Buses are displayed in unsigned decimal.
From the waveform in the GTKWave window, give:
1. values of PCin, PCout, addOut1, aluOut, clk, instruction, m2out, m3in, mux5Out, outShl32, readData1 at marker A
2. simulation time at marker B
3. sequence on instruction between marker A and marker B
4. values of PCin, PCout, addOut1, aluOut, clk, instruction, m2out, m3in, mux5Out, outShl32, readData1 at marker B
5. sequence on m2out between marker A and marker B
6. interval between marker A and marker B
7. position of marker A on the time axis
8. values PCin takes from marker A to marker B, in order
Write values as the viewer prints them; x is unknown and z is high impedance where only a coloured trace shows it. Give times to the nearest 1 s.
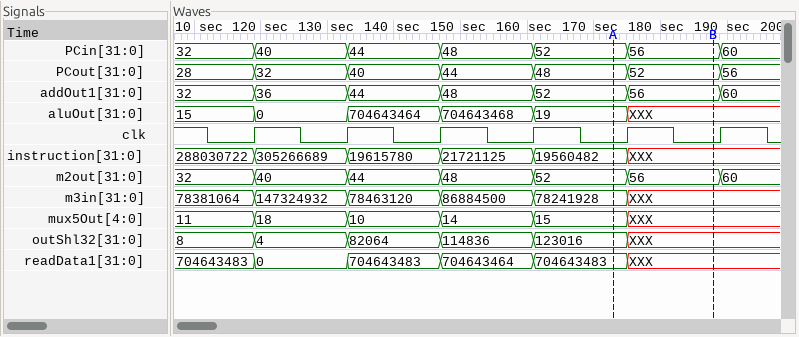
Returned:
PCin=52, PCout=48, addOut1=52, aluOut=19, clk=0, instruction=19560482, m2out=52, m3in=78241928, mux5Out=15, outShl32=123016, readData1=704643483
188 s
19560482, XXX
PCin=56, PCout=52, addOut1=56, aluOut=XXX, clk=0, instruction=XXX, m2out=56, m3in=XXX, mux5Out=XXX, outShl32=XXX, readData1=XXX
52, 56
15 s
173 s
52, 56
